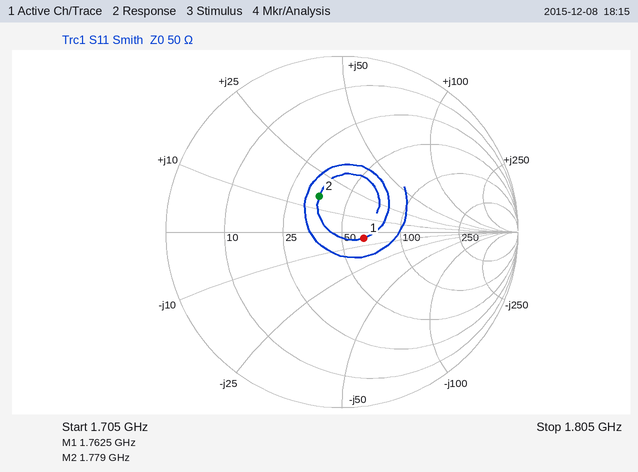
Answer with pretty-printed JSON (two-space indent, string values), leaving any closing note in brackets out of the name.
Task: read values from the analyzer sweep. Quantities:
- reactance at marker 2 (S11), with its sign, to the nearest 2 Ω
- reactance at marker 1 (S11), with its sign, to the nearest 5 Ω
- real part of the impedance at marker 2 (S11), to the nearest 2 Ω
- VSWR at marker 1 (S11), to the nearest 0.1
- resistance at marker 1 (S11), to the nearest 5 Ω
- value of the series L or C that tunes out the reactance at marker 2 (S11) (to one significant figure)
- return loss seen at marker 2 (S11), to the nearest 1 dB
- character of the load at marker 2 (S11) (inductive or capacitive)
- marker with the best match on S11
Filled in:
{
  "reactance at marker 2 (S11), with its sign, to the nearest 2 Ω": "+16 Ω",
  "reactance at marker 1 (S11), with its sign, to the nearest 5 Ω": "-5 Ω",
  "real part of the impedance at marker 2 (S11), to the nearest 2 Ω": "36 Ω",
  "VSWR at marker 1 (S11), to the nearest 0.1": "1.3",
  "resistance at marker 1 (S11), to the nearest 5 Ω": "65 Ω",
  "value of the series L or C that tunes out the reactance at marker 2 (S11)": "6 pF",
  "return loss seen at marker 2 (S11), to the nearest 1 dB": "12 dB",
  "character of the load at marker 2 (S11)": "inductive",
  "marker with the best match on S11": "marker 1"
}
